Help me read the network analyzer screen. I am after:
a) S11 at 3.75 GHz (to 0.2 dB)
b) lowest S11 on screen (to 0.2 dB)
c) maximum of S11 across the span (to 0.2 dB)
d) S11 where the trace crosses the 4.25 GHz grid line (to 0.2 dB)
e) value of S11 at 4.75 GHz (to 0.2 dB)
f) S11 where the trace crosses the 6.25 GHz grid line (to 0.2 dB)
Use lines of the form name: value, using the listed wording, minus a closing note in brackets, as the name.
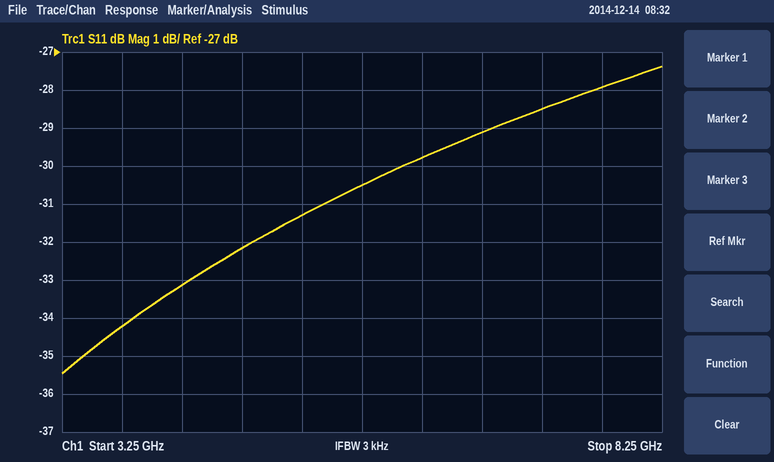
S11 at 3.75 GHz: -34.2 dB
lowest S11 on screen: -35.4 dB
maximum of S11 across the span: -27.4 dB
S11 where the trace crosses the 4.25 GHz grid line: -33.2 dB
value of S11 at 4.75 GHz: -32.2 dB
S11 where the trace crosses the 6.25 GHz grid line: -29.8 dB
